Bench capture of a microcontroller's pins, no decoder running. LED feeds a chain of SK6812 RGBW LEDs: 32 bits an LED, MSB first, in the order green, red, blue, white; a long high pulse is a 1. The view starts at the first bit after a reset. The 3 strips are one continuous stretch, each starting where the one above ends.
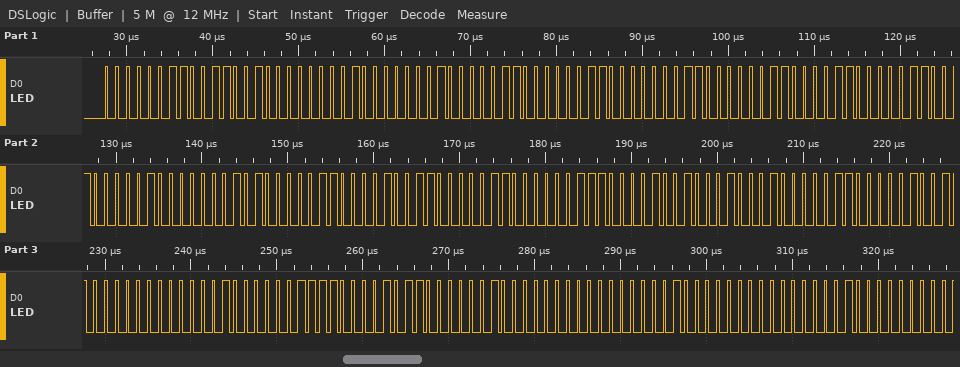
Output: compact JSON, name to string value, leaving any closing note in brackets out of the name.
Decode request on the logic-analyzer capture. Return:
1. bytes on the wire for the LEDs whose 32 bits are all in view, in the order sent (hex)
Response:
{"bytes on the wire for the LEDs whose 32 bits are all in view, in the order sent": "03 32 01 01 06 06 03 03 0C 19 04 05 06 13 06 07 09 11 06 09 00 04 0F 0B 02 00 01 00"}
